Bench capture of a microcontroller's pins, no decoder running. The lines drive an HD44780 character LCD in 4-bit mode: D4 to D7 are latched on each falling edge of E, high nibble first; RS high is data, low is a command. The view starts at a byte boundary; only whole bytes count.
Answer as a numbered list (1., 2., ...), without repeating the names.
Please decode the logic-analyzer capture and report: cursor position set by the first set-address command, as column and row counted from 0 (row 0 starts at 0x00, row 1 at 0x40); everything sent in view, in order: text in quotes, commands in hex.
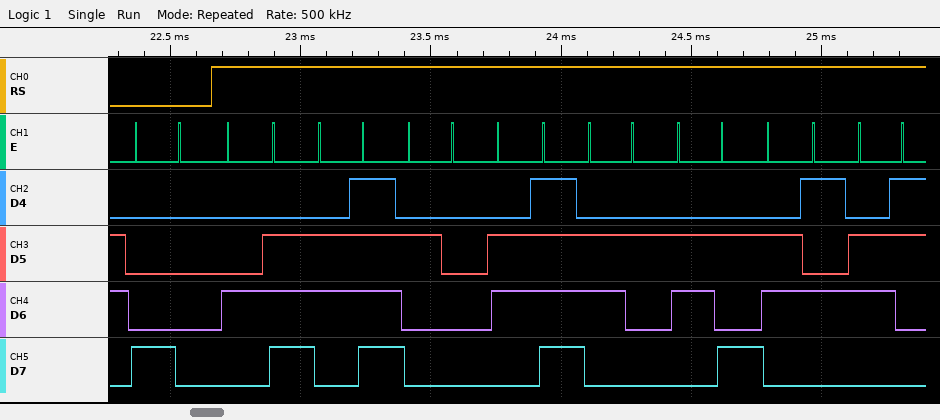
1. column 0, row 0
2. 0x80 "No objec"
